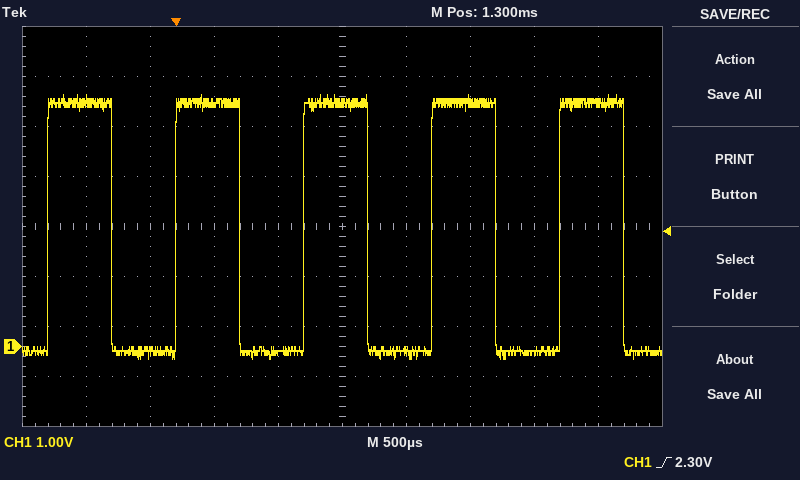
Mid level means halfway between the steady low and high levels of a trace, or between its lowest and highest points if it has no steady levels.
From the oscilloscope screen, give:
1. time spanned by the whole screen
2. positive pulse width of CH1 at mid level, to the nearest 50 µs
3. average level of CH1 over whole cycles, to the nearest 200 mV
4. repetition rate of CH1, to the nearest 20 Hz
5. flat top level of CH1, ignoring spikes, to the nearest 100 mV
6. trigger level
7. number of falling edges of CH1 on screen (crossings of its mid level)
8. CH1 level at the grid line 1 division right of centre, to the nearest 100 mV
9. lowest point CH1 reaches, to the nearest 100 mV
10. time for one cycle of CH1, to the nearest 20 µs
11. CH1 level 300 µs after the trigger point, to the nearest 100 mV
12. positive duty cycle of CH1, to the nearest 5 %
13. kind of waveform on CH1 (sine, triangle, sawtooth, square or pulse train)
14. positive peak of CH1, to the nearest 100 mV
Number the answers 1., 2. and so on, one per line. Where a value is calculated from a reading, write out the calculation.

1. 5 ms
2. 500 µs
3. -200 mV + 0.5 × (4.9 V − (-200 mV)) ≈ 2.4 V
4. 1 / 1.00 ms ≈ 1.00 kHz
5. 4.9 V
6. 2.30 V
7. 5
8. -100 mV
9. -200 mV
10. 1.00 ms
11. 4.9 V
12. 500 µs / 1.00 ms ≈ 50 %
13. square
14. 5.0 V
